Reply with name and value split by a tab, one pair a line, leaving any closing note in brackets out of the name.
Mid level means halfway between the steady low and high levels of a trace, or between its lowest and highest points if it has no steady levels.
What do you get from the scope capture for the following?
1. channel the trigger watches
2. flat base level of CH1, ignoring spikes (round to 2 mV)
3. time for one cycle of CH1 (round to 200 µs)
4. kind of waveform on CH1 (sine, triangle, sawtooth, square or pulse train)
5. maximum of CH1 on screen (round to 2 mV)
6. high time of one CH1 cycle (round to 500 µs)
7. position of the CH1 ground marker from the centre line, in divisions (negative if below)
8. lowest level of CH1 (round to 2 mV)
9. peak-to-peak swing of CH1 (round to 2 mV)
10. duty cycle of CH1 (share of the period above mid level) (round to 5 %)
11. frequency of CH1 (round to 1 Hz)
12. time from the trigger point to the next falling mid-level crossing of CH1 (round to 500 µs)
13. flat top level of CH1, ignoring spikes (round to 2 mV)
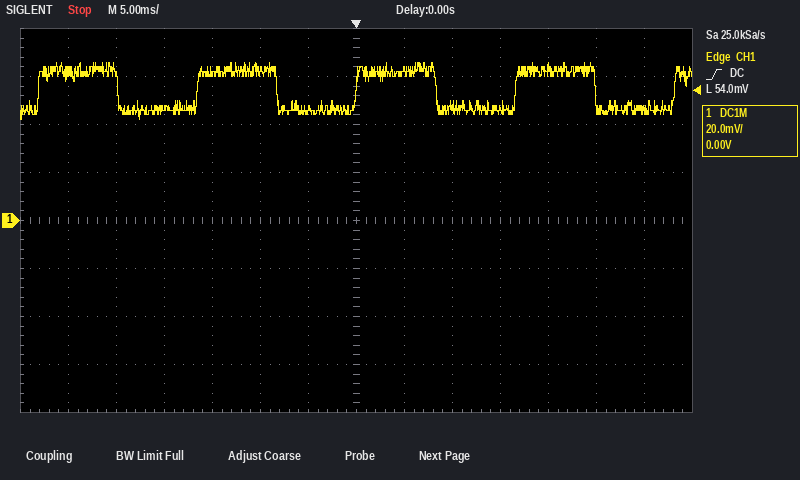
channel the trigger watches	CH1
flat base level of CH1, ignoring spikes	46 mV
time for one cycle of CH1	16.6 ms
kind of waveform on CH1	square
maximum of CH1 on screen	66 mV
high time of one CH1 cycle	8.5 ms
position of the CH1 ground marker from the centre line, in divisions	0.0 div
lowest level of CH1	42 mV
peak-to-peak swing of CH1	24 mV
duty cycle of CH1 (share of the period above mid level)	50 %
frequency of CH1	60 Hz
time from the trigger point to the next falling mid-level crossing of CH1	8.5 ms
flat top level of CH1, ignoring spikes	62 mV
